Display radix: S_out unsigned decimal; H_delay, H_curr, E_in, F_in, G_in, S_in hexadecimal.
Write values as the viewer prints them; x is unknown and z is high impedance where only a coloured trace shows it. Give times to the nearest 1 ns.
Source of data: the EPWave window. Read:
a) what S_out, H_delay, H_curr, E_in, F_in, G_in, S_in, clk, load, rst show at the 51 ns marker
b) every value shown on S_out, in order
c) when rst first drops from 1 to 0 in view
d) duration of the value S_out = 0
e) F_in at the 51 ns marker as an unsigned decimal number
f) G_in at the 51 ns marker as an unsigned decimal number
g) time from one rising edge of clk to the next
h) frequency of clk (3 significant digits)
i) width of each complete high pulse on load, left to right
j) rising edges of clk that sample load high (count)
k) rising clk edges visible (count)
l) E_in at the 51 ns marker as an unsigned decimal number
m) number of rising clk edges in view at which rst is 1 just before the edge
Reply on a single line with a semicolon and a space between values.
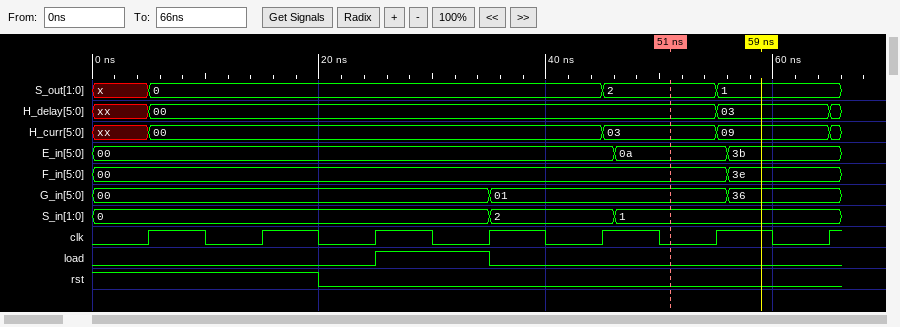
S_out=2, H_delay=00, H_curr=03, E_in=0a, F_in=00, G_in=01, S_in=1, clk=0, load=0, rst=0; x, 0, 2, 1; 20 ns; 40 ns; 0; 1; 10 ns; 100 MHz; 10 ns; 1; 7; 10; 2
